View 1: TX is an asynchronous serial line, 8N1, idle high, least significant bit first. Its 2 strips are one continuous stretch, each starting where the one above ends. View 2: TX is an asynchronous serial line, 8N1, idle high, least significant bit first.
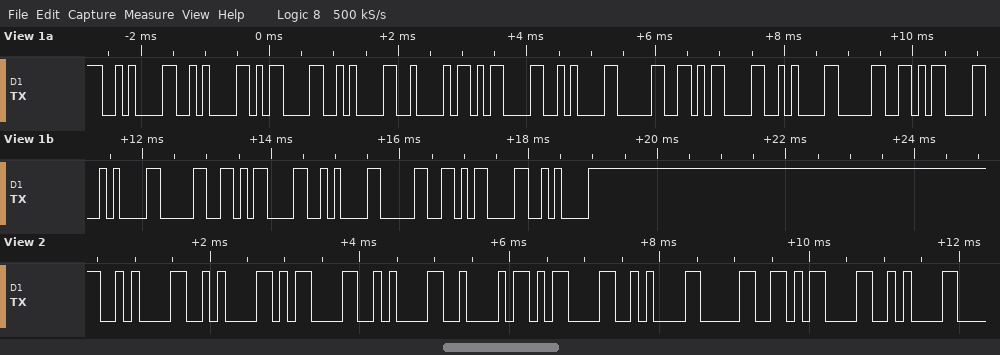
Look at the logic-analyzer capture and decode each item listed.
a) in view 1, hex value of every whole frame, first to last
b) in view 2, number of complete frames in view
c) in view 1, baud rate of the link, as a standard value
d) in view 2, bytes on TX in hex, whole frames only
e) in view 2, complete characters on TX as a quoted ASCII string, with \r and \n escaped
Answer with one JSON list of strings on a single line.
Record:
["0A 0A 0D 0A 42 0D 0A 30 0D 0A 30 0D 0A 30 0D 0A 30 0D 0A", "10", "9600 baud", "0x0A 0x0A 0x0D 0x0A 0x42 0x0D 0x0A 0x30 0x0D 0x0A", "\"\\n\\n\\r\\nB\\r\\n0\\r\\n\""]
